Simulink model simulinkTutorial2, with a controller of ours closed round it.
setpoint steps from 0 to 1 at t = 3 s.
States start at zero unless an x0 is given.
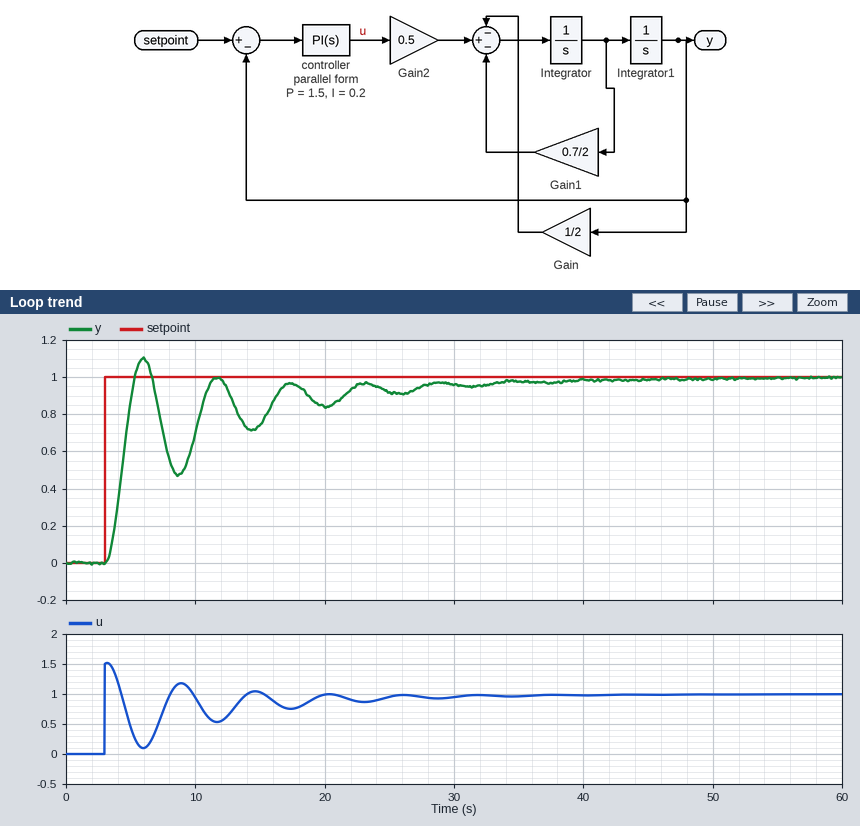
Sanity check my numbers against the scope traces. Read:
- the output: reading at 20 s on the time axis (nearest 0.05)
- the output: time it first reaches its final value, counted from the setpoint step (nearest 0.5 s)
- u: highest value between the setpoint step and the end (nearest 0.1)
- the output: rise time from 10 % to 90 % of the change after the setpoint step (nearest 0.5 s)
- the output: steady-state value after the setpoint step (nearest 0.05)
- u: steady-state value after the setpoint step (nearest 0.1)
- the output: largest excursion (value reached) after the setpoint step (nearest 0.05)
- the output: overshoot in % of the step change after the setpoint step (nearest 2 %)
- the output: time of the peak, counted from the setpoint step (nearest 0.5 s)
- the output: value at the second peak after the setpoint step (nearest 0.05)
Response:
0.85
2.5 s
1.5
1.5 s
1.00
1.0
1.10
10 %
3.0 s
1.00
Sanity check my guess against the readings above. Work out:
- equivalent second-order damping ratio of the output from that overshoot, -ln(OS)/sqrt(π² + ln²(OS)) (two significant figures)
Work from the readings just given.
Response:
0.59
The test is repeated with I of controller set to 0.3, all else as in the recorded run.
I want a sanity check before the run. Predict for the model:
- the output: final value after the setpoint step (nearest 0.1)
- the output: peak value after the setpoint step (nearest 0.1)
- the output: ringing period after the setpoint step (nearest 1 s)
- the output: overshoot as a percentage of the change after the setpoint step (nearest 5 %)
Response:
1.0
1.2
6 s
15 %
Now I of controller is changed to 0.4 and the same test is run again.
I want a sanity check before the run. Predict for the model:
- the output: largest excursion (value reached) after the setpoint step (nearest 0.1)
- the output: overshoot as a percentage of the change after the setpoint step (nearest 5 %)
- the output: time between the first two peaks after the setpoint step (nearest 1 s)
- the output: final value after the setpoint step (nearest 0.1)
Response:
1.2
25 %
6 s
1.0
